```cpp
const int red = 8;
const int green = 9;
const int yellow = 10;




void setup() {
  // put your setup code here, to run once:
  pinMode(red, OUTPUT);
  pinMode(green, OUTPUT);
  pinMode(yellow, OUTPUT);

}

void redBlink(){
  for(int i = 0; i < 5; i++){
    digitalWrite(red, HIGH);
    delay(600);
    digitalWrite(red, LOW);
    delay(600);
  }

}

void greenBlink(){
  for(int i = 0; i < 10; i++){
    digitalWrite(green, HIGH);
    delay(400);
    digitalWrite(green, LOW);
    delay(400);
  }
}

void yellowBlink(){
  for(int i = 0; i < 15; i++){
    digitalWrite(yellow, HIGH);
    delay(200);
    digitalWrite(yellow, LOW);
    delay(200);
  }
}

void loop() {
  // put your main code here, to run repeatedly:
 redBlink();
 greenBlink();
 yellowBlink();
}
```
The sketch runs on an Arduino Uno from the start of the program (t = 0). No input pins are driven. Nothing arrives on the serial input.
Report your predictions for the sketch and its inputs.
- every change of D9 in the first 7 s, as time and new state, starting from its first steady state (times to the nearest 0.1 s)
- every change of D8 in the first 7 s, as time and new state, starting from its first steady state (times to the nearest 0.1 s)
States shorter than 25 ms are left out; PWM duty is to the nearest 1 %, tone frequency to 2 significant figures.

0 s low; 6 s high; 6.4 s low; 6.8 s high
0 s high; 0.6 s low; 1.2 s high; 1.8 s low; 2.4 s high; 3 s low; 3.6 s high; 4.2 s low; 4.8 s high; 5.4 s low
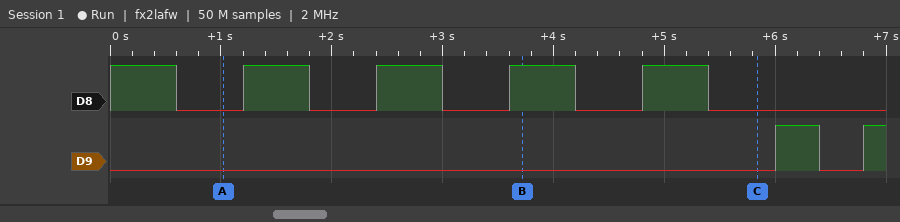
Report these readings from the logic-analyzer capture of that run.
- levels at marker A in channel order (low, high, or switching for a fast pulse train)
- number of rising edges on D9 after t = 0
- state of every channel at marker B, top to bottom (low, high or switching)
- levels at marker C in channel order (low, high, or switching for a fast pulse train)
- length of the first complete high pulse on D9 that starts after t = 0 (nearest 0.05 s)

D8 low, D9 low
2
D8 high, D9 low
D8 low, D9 low
0.40 s
